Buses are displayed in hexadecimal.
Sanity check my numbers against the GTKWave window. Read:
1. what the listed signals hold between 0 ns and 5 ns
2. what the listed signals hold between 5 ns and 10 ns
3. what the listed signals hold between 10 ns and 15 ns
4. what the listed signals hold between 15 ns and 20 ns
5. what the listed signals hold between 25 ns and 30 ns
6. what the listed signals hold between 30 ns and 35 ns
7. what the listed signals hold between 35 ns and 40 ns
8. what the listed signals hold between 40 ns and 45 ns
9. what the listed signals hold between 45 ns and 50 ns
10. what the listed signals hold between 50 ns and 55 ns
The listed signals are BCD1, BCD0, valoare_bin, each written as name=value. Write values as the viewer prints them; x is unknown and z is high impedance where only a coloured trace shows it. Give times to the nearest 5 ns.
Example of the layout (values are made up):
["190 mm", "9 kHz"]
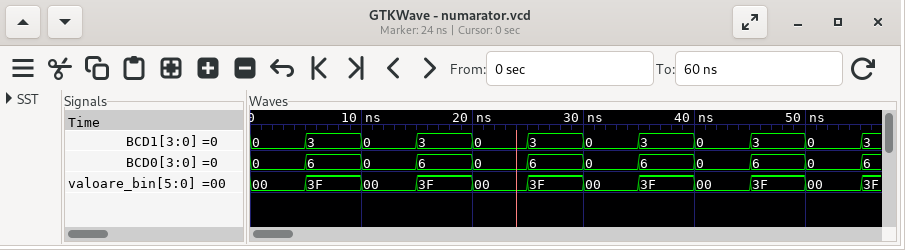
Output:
["BCD1=0, BCD0=0, valoare_bin=00", "BCD1=3, BCD0=6, valoare_bin=3F", "BCD1=0, BCD0=0, valoare_bin=00", "BCD1=3, BCD0=6, valoare_bin=3F", "BCD1=3, BCD0=6, valoare_bin=3F", "BCD1=0, BCD0=0, valoare_bin=00", "BCD1=3, BCD0=6, valoare_bin=3F", "BCD1=0, BCD0=0, valoare_bin=00", "BCD1=3, BCD0=6, valoare_bin=3F", "BCD1=0, BCD0=0, valoare_bin=00"]
